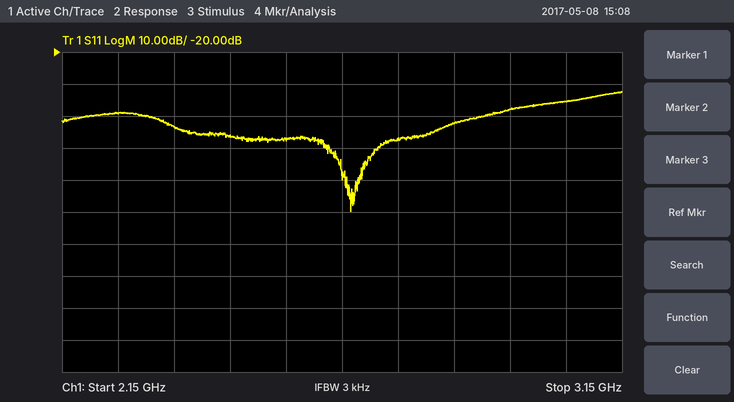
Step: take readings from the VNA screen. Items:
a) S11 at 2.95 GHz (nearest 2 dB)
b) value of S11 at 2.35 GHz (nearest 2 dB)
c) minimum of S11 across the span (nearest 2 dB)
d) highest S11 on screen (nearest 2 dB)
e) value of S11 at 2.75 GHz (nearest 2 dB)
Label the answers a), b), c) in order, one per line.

a) -38 dB
b) -44 dB
c) -70 dB
d) -32 dB
e) -48 dB
